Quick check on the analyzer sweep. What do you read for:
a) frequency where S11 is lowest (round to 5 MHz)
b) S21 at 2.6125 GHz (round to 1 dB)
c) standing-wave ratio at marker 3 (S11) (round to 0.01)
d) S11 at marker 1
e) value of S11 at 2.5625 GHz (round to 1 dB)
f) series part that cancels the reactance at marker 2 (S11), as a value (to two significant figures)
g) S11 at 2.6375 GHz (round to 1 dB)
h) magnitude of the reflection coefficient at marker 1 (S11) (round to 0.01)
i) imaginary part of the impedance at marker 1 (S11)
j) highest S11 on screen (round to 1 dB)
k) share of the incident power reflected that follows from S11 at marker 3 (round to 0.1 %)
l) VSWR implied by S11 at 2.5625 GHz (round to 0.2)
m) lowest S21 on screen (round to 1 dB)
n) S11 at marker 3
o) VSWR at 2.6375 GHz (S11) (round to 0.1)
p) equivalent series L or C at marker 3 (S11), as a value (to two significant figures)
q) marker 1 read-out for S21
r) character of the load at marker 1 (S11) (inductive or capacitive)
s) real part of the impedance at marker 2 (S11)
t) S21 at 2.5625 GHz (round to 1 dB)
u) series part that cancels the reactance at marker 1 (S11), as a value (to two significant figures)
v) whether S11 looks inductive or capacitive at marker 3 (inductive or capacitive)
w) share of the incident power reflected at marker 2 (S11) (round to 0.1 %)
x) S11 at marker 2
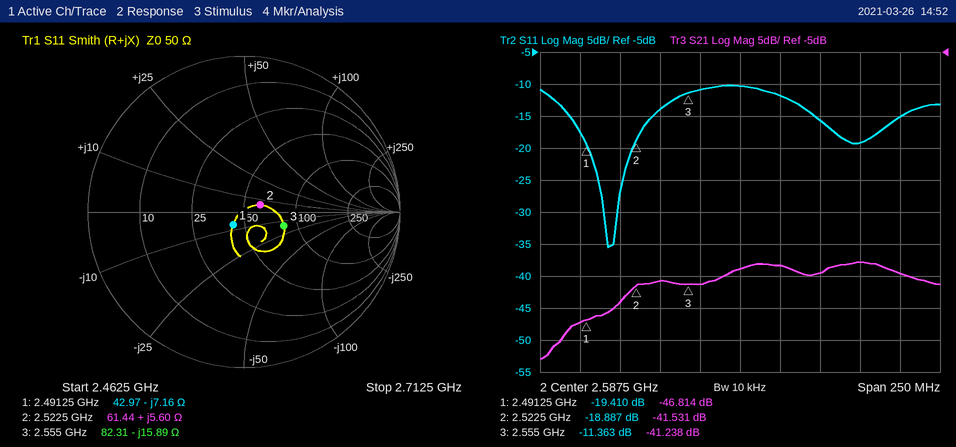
2.505 GHz
-38 dB
1.74
-19.410 dB
-11 dB
11 pF
-16 dB
0.11
-7.16 Ω
-10 dB
7.3 %
1.8
-53 dB
-11.363 dB
1.4
3.9 pF
-46.814 dB
capacitive
61.44 Ω
-41 dB
460 pH
capacitive
1.3 %
-18.887 dB
